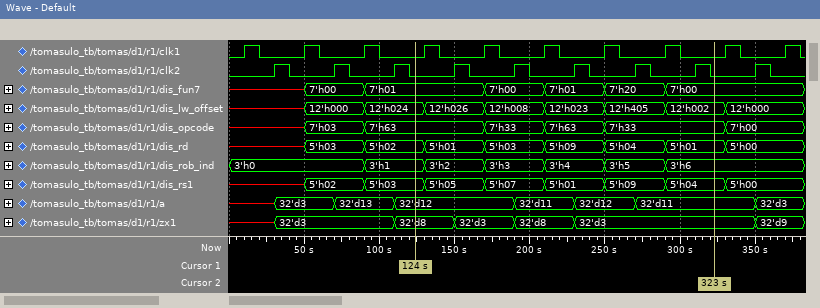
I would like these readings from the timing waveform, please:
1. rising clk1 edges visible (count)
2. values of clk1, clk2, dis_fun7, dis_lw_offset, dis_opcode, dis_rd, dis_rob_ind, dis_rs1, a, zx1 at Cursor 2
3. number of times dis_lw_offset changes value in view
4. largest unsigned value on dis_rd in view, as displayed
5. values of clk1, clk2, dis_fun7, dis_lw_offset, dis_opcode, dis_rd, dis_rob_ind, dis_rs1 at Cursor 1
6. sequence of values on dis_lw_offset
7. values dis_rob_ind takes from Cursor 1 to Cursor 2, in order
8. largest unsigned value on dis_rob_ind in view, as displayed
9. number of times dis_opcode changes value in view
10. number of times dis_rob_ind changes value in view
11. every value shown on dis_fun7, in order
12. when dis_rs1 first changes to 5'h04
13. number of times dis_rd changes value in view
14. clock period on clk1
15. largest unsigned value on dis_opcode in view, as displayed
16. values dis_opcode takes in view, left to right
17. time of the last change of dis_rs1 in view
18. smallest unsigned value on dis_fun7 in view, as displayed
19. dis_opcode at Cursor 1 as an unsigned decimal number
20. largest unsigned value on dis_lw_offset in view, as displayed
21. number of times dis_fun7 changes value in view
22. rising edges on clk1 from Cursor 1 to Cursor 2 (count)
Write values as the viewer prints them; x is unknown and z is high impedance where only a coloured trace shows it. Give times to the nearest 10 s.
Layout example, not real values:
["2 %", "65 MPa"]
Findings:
["10", "clk1=0, clk2=0, dis_fun7=7'h00, dis_lw_offset=12'h002, dis_opcode=7'h33, dis_rd=5'h01, dis_rob_ind=3'h6, dis_rs1=5'h04, a=32'd11, zx1=32'd3", "8", "5'h09", "clk1=0, clk2=0, dis_fun7=7'h01, dis_lw_offset=12'h024, dis_opcode=7'h63, dis_rd=5'h02, dis_rob_ind=3'h1, dis_rs1=5'h03", "x, 12'h000, 12'h024, 12'h026, 12'h008, 12'h023, 12'h405, 12'h002, 12'h000", "3'h1, 3'h2, 3'h3, 3'h4, 3'h5, 3'h6", "3'h6", "6", "6", "x, 7'h00, 7'h01, 7'h00, 7'h01, 7'h20, 7'h00", "290 s", "8", "40 s", "7'h63", "x, 7'h03, 7'h63, 7'h33, 7'h63, 7'h33, 7'h00", "330 s", "7'h00", "99", "12'h405", "6", "5"]
